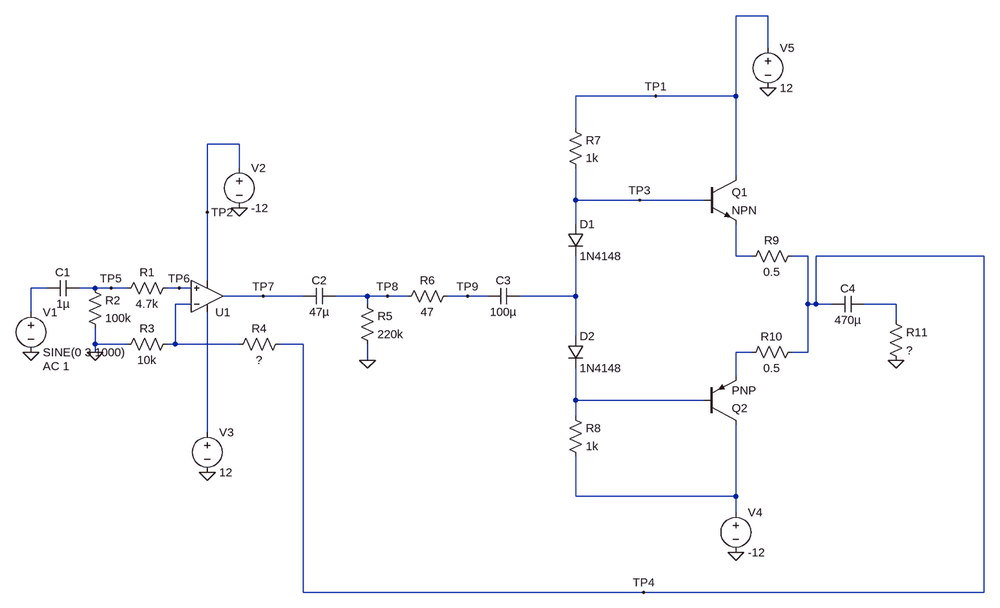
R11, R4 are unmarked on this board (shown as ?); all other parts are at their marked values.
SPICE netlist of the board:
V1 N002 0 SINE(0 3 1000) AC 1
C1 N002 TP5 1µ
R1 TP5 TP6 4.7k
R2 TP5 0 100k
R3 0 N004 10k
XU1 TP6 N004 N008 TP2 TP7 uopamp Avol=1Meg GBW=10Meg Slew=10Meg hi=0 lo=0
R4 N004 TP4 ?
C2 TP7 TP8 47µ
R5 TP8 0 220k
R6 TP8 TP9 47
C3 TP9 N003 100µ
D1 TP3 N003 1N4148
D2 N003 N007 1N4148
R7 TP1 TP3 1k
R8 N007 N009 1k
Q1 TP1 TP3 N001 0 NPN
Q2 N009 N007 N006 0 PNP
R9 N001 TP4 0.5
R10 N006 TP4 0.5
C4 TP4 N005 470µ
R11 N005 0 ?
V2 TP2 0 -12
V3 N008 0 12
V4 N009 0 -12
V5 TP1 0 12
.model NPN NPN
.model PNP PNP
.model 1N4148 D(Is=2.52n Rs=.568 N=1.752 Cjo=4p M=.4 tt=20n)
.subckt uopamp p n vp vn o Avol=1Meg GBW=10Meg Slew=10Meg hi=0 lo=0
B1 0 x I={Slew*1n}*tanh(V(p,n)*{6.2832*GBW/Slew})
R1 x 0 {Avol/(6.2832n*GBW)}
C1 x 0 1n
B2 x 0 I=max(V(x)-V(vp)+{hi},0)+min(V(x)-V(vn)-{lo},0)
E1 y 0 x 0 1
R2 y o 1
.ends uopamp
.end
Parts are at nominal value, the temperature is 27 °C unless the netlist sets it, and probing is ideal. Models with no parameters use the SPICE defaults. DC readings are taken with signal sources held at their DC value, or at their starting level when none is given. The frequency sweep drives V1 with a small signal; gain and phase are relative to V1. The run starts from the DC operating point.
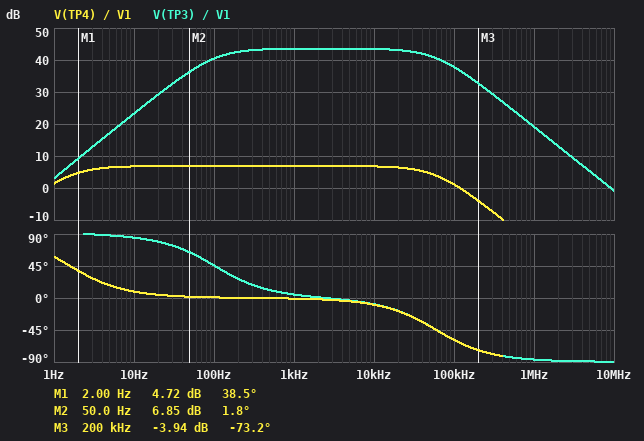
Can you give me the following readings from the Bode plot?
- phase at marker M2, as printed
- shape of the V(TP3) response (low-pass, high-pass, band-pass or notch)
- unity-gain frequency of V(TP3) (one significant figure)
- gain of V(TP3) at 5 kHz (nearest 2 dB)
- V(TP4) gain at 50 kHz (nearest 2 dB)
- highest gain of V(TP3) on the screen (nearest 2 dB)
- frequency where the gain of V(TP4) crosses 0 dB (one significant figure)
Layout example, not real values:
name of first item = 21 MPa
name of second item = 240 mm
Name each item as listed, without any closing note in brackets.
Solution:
phase at marker M2, as printed = 1.8 deg
shape of the V(TP3) response = band-pass
unity-gain frequency of V(TP3) = 9 MHz
gain of V(TP3) at 5 kHz = 44 dB
V(TP4) gain at 50 kHz = 4 dB
highest gain of V(TP3) on the screen = 44 dB
frequency where the gain of V(TP4) crosses 0 dB = 100 kHz
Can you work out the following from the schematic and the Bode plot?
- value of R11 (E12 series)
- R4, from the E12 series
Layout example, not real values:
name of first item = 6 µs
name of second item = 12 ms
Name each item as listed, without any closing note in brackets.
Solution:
value of R11 = 3.3 Ω
R4, from the E12 series = 12 kΩ
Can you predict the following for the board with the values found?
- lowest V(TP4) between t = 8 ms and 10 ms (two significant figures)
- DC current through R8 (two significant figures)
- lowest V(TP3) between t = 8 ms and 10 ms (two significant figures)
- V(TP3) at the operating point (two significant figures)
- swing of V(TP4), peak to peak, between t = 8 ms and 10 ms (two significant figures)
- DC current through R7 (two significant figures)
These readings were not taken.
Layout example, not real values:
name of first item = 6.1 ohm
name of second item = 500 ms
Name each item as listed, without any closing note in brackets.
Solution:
lowest V(TP4) between t = 8 ms and 10 ms = -2.9 V
DC current through R8 = 11 mA
lowest V(TP3) between t = 8 ms and 10 ms = -10 V
V(TP3) at the operating point = 700 mV
swing of V(TP4), peak to peak, between t = 8 ms and 10 ms = 5.8 V
DC current through R7 = 11 mA
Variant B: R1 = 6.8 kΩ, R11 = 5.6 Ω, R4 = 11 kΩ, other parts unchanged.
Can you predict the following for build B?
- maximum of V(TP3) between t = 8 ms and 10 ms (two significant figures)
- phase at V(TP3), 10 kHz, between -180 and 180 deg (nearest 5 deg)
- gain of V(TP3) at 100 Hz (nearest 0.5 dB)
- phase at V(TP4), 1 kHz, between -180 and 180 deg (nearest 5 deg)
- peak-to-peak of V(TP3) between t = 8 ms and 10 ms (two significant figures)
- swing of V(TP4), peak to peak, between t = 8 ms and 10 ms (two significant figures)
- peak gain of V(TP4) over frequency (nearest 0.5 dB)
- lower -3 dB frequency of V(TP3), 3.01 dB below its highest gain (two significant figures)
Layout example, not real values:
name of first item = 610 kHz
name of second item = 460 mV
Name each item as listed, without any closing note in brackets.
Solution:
maximum of V(TP3) between t = 8 ms and 10 ms = 5.3 V
phase at V(TP3), 10 kHz, between -180 and 180 deg = -5 deg
gain of V(TP3) at 100 Hz = 37.5 dB
phase at V(TP4), 1 kHz, between -180 and 180 deg = 0 deg
peak-to-peak of V(TP3) between t = 8 ms and 10 ms = 16 V
swing of V(TP4), peak to peak, between t = 8 ms and 10 ms = 8.0 V
peak gain of V(TP4) over frequency = 6.5 dB
lower -3 dB frequency of V(TP3), 3.01 dB below its highest gain = 60 Hz
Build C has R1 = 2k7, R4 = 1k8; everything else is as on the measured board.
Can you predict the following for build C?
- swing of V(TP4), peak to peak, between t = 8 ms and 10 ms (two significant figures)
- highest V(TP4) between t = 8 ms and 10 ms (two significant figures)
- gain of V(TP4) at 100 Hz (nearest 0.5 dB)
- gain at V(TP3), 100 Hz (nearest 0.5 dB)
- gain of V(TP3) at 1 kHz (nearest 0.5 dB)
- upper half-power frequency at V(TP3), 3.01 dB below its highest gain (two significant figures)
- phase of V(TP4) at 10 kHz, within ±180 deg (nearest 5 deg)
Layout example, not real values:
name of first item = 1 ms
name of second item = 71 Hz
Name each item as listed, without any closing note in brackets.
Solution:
swing of V(TP4), peak to peak, between t = 8 ms and 10 ms = 5.6 V
highest V(TP4) between t = 8 ms and 10 ms = 2.8 V
gain of V(TP4) at 100 Hz = 1.5 dB
gain at V(TP3), 100 Hz = 35.0 dB
gain of V(TP3) at 1 kHz = 38.0 dB
upper half-power frequency at V(TP3), 3.01 dB below its highest gain = 110 kHz
phase of V(TP4) at 10 kHz, within ±180 deg = -5 deg
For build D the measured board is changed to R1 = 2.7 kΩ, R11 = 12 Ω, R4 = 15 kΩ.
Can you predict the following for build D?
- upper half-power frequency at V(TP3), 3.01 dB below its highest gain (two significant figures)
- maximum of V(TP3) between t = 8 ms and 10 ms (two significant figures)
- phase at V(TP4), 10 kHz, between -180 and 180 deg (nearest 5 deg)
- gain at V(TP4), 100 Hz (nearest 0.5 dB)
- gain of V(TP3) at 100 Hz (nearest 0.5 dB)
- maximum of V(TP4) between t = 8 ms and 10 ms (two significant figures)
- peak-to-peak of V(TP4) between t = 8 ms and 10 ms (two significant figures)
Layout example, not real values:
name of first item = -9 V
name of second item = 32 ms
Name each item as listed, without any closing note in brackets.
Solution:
upper half-power frequency at V(TP3), 3.01 dB below its highest gain = 190 kHz
maximum of V(TP3) between t = 8 ms and 10 ms = 7.2 V
phase at V(TP4), 10 kHz, between -180 and 180 deg = -5 deg
gain at V(TP4), 100 Hz = 8.0 dB
gain of V(TP3) at 100 Hz = 33.5 dB
maximum of V(TP4) between t = 8 ms and 10 ms = 6.0 V
peak-to-peak of V(TP4) between t = 8 ms and 10 ms = 12 V
